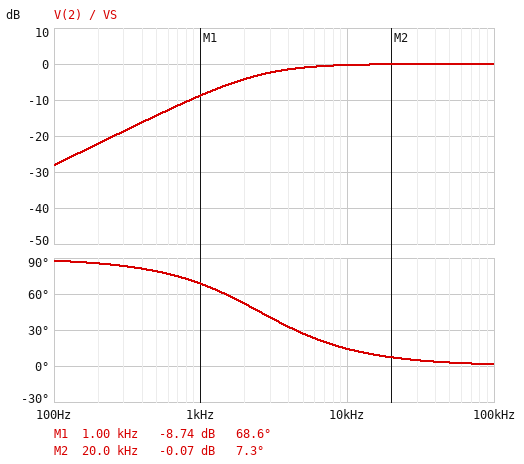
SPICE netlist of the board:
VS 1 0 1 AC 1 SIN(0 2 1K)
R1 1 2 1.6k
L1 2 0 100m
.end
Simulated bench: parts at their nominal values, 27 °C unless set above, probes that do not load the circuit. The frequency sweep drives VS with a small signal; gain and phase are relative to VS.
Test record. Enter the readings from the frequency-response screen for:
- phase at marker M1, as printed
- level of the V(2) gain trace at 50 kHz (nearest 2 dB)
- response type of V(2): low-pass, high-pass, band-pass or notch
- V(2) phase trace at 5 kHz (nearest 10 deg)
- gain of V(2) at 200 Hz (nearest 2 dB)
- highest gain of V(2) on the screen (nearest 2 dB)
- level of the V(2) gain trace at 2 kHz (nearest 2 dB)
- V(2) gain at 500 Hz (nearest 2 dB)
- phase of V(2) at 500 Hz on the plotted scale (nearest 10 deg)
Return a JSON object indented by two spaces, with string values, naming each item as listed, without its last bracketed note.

{
  "phase at marker M1, as printed": "68.6 deg",
  "level of the V(2) gain trace at 50 kHz": "0 dB",
  "response type of V(2): low-pass, high-pass, band-pass or notch": "high-pass",
  "V(2) phase trace at 5 kHz": "30 deg",
  "gain of V(2) at 200 Hz": "-22 dB",
  "highest gain of V(2) on the screen": "0 dB",
  "level of the V(2) gain trace at 2 kHz": "-4 dB",
  "V(2) gain at 500 Hz": "-14 dB",
  "phase of V(2) at 500 Hz on the plotted scale": "80 deg"
}
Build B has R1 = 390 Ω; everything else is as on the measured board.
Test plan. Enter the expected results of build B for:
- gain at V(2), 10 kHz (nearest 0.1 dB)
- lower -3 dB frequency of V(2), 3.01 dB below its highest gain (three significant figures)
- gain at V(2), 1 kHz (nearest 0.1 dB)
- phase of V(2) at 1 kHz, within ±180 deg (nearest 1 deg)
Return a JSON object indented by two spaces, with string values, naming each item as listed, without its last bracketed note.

{
  "gain at V(2), 10 kHz": "0 dB",
  "lower -3 dB frequency of V(2), 3.01 dB below its highest gain": "621 Hz",
  "gain at V(2), 1 kHz": "-1.4 dB",
  "phase of V(2) at 1 kHz, within ±180 deg": "32 deg"
}
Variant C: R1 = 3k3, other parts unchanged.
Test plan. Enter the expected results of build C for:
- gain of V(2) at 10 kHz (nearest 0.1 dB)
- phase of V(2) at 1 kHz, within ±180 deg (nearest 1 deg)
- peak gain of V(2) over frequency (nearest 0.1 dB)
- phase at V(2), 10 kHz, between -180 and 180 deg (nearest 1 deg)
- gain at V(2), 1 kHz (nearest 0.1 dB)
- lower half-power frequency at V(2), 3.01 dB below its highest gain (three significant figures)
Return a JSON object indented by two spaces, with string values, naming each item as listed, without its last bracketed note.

{
  "gain of V(2) at 10 kHz": "-1.1 dB",
  "phase of V(2) at 1 kHz, within ±180 deg": "79 deg",
  "peak gain of V(2) over frequency": "0 dB",
  "phase at V(2), 10 kHz, between -180 and 180 deg": "28 deg",
  "gain at V(2), 1 kHz": "-14.6 dB",
  "lower half-power frequency at V(2), 3.01 dB below its highest gain": "5.25 kHz"
}
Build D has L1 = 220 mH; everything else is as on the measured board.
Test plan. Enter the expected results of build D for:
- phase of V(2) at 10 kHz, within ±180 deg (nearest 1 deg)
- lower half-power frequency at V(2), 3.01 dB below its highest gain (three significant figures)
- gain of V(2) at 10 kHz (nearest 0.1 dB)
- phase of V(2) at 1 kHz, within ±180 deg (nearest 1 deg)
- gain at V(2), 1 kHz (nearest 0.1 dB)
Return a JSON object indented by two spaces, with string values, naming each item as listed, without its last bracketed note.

{
  "phase of V(2) at 10 kHz, within ±180 deg": "7 deg",
  "lower half-power frequency at V(2), 3.01 dB below its highest gain": "1.16 kHz",
  "gain of V(2) at 10 kHz": "-0.1 dB",
  "phase of V(2) at 1 kHz, within ±180 deg": "49 deg",
  "gain at V(2), 1 kHz": "-3.7 dB"
}
